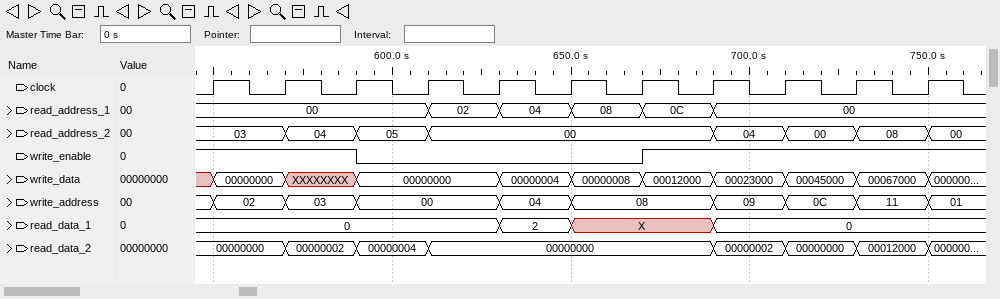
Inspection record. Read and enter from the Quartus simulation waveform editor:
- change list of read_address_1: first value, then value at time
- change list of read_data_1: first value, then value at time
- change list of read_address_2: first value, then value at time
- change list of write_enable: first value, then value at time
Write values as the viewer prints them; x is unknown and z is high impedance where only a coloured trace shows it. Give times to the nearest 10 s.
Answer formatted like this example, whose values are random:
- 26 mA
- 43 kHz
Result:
- 00, 02 at 610 s, 04 at 630 s, 08 at 650 s, 0C at 670 s, 00 at 690 s
- 0, 2 at 630 s, X at 650 s, 0 at 690 s
- 03, 04 at 570 s, 05 at 590 s, 00 at 610 s, 04 at 690 s, 00 at 710 s, 08 at 730 s, 00 at 750 s
- 1, 0 at 590 s, 1 at 670 s
